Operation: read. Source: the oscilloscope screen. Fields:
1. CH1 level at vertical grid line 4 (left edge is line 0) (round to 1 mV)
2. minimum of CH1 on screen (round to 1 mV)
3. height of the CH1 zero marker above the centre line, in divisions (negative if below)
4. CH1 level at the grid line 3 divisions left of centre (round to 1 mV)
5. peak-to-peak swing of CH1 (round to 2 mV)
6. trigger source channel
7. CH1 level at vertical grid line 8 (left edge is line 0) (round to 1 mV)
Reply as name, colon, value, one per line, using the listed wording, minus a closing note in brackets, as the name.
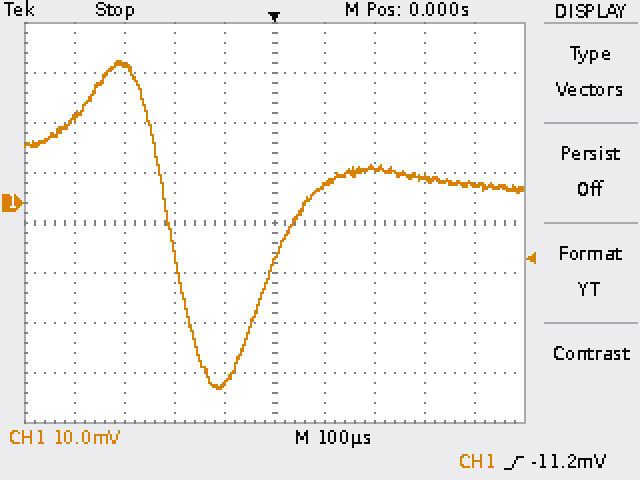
CH1 level at vertical grid line 4 (left edge is line 0): -36 mV
minimum of CH1 on screen: -37 mV
height of the CH1 zero marker above the centre line, in divisions: +0.4 div
CH1 level at the grid line 3 divisions left of centre: 28 mV
peak-to-peak swing of CH1: 66 mV
trigger source channel: CH1
CH1 level at vertical grid line 8 (left edge is line 0): 5 mV
